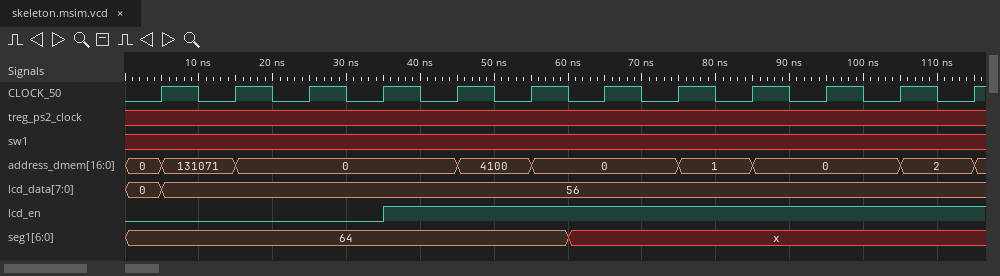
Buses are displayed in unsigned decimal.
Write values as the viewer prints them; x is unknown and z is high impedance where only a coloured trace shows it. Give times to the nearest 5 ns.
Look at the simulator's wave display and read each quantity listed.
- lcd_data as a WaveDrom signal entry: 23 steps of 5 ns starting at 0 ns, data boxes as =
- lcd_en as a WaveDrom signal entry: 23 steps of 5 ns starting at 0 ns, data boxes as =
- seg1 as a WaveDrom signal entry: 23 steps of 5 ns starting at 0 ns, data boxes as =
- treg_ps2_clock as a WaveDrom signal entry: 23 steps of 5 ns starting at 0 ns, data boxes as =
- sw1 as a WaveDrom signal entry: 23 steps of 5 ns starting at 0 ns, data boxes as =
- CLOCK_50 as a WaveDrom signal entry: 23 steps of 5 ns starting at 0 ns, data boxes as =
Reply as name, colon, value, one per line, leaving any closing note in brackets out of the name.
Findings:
lcd_data as a WaveDrom signal entry: 23 steps of 5 ns starting at 0 ns, data boxes as =: {name: 'lcd_data', wave: '==.....................', data: '0 56'}
lcd_en as a WaveDrom signal entry: 23 steps of 5 ns starting at 0 ns, data boxes as =: {name: 'lcd_en', wave: '0......1...............'}
seg1 as a WaveDrom signal entry: 23 steps of 5 ns starting at 0 ns, data boxes as =: {name: 'seg1', wave: '=...........x..........', data: '64'}
treg_ps2_clock as a WaveDrom signal entry: 23 steps of 5 ns starting at 0 ns, data boxes as =: {name: 'treg_ps2_clock', wave: 'x......................'}
sw1 as a WaveDrom signal entry: 23 steps of 5 ns starting at 0 ns, data boxes as =: {name: 'sw1', wave: 'x......................'}
CLOCK_50 as a WaveDrom signal entry: 23 steps of 5 ns starting at 0 ns, data boxes as =: {name: 'CLOCK_50', wave: '01010101010101010101010'}
